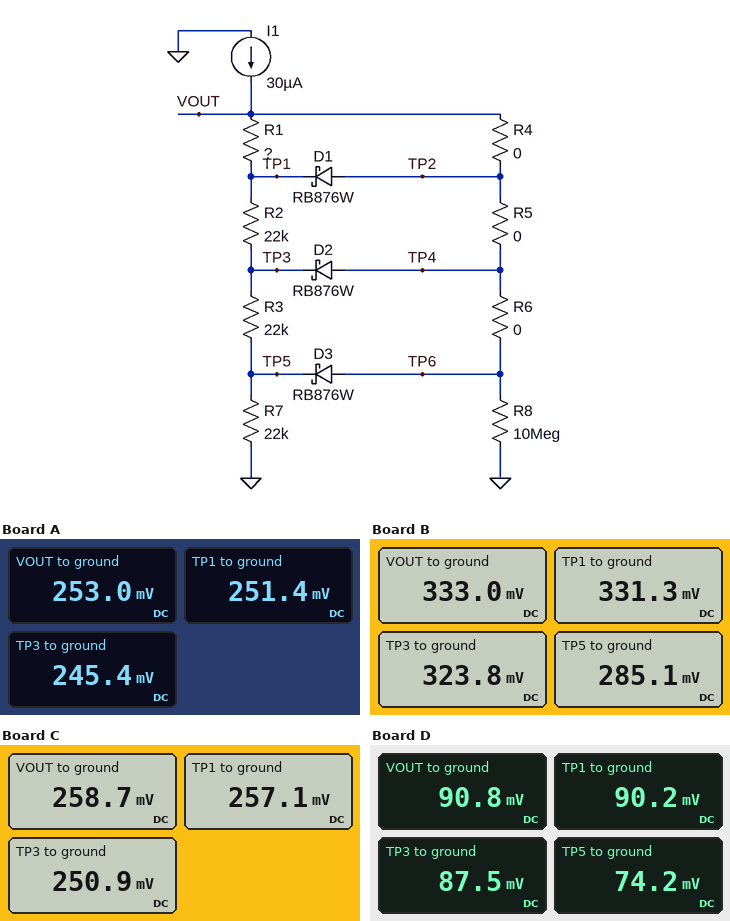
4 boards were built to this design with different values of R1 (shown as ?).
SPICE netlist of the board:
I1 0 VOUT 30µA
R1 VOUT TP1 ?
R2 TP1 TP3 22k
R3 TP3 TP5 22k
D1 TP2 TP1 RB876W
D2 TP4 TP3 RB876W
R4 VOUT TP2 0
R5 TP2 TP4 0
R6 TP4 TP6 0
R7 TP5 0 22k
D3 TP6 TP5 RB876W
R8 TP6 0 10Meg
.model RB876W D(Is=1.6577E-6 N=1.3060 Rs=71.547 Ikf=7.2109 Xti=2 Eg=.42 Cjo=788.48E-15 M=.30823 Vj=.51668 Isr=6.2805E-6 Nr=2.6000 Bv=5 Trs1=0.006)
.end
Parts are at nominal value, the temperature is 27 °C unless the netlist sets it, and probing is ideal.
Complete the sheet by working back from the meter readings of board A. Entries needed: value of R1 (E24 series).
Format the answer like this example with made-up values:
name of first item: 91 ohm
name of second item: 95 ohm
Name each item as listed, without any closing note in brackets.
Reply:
value of R1: 36 kΩ
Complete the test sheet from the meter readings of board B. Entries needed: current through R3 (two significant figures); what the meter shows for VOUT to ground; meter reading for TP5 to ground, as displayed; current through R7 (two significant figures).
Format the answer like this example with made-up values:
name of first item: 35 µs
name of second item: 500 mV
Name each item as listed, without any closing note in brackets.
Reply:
current through R3: 1.8 µA
what the meter shows for VOUT to ground: 333.0 mV
meter reading for TP5 to ground, as displayed: 285.1 mV
current through R7: 13 µA
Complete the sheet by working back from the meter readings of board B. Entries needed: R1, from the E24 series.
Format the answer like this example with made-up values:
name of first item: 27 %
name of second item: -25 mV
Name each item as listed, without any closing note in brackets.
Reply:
R1, from the E24 series: 18 kΩ
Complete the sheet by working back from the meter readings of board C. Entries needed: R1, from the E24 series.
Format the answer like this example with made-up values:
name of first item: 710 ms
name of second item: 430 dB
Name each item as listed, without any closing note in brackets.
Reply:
R1, from the E24 series: 33 kΩ
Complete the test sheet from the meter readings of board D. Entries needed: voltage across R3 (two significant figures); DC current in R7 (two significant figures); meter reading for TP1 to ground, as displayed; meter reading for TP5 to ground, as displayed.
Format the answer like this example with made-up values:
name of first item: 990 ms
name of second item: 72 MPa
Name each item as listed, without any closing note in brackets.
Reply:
voltage across R3: 13 mV
DC current in R7: 3.4 µA
meter reading for TP1 to ground, as displayed: 90.2 mV
meter reading for TP5 to ground, as displayed: 74.2 mV
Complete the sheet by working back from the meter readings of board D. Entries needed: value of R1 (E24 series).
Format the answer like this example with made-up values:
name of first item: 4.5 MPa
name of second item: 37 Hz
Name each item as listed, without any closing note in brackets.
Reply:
value of R1: 16 kΩ
